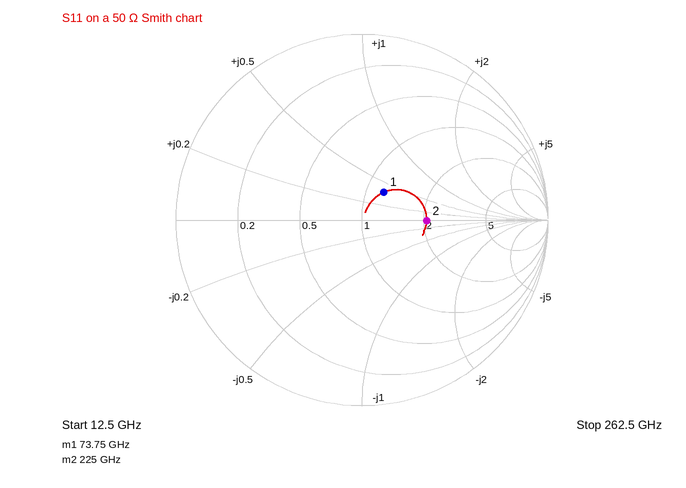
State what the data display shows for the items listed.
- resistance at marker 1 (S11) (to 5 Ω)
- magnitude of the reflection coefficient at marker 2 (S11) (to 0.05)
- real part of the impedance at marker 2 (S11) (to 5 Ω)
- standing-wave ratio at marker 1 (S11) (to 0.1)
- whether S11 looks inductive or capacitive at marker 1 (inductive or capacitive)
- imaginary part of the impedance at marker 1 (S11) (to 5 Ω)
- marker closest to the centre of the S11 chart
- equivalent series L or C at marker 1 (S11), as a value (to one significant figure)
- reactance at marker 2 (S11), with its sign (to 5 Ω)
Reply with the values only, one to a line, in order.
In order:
60 Ω
0.35
105 Ω
1.5
inductive
+20 Ω
marker 1
40 pH
0 Ω
